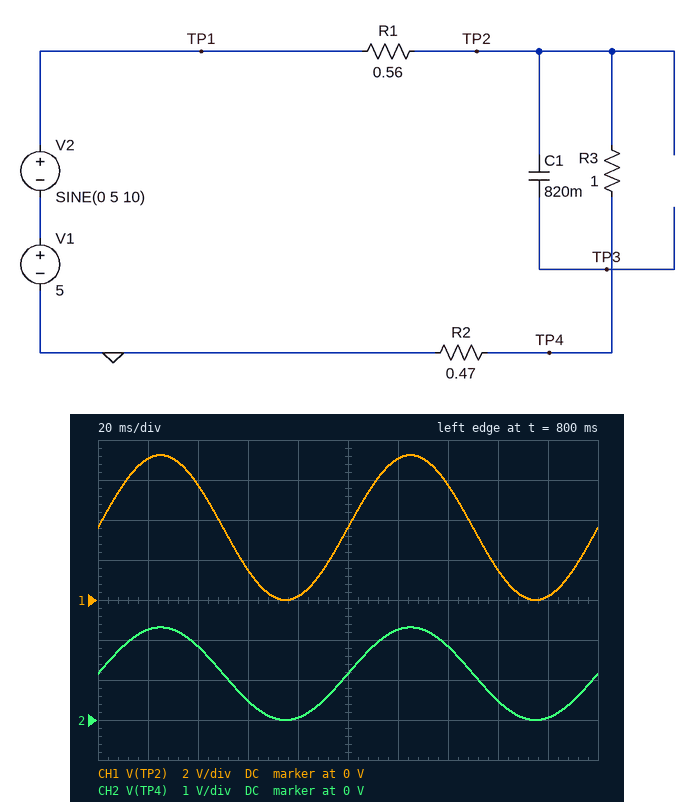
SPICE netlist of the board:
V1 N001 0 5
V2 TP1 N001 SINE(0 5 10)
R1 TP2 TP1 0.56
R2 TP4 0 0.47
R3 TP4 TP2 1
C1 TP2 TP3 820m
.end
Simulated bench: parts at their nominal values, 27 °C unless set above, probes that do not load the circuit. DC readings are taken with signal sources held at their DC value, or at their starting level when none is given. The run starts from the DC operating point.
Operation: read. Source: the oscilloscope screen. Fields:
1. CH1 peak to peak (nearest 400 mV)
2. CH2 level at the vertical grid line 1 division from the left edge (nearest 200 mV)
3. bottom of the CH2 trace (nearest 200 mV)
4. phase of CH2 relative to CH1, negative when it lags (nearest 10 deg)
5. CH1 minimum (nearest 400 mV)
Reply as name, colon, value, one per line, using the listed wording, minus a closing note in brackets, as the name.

CH1 peak to peak: 7.2 V
CH2 level at the vertical grid line 1 division from the left edge: 2.2 V
bottom of the CH2 trace: 0 V
phase of CH2 relative to CH1, negative when it lags: 0 deg
CH1 minimum: 0 V
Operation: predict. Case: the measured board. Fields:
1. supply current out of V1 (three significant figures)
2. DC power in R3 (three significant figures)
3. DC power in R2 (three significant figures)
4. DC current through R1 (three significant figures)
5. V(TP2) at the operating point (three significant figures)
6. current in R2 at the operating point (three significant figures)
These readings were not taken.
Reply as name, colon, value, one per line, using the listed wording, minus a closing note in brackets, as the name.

supply current out of V1: 2.46 A
DC power in R3: 6.07 W
DC power in R2: 2.85 W
DC current through R1: 2.46 A
V(TP2) at the operating point: 3.62 V
current in R2 at the operating point: 2.46 A
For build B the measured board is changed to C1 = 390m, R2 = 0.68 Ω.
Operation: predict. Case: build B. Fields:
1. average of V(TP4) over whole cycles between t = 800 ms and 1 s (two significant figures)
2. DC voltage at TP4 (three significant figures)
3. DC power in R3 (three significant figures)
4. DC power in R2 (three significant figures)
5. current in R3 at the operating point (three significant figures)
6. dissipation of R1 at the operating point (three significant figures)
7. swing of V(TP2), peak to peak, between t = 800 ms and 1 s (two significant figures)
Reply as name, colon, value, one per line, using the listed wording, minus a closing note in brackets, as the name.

average of V(TP4) over whole cycles between t = 800 ms and 1 s: 1.5 V
DC voltage at TP4: 1.52 V
DC power in R3: 4.98 W
DC power in R2: 3.39 W
current in R3 at the operating point: 2.23 A
dissipation of R1 at the operating point: 2.79 W
swing of V(TP2), peak to peak, between t = 800 ms and 1 s: 7.5 V
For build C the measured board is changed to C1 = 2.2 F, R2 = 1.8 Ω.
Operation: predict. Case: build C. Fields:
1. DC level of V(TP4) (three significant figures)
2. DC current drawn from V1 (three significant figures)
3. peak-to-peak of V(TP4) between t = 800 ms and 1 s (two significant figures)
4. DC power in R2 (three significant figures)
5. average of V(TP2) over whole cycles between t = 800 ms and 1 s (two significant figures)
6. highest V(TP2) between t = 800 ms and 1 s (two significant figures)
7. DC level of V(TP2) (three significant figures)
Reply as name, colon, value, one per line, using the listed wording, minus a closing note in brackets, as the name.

DC level of V(TP4): 2.68 V
DC current drawn from V1: 1.49 A
peak-to-peak of V(TP4) between t = 800 ms and 1 s: 5.4 V
DC power in R2: 3.99 W
average of V(TP2) over whole cycles between t = 800 ms and 1 s: 4.2 V
highest V(TP2) between t = 800 ms and 1 s: 8.3 V
DC level of V(TP2): 4.17 V
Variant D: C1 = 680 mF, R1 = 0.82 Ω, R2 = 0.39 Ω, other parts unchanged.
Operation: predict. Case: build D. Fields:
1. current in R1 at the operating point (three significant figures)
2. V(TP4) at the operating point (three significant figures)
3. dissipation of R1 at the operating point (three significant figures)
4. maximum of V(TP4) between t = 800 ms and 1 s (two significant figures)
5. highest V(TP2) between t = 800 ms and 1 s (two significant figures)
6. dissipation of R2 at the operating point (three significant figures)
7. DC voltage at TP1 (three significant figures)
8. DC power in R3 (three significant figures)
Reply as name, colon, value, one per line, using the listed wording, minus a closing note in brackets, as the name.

current in R1 at the operating point: 2.26 A
V(TP4) at the operating point: 882 mV
dissipation of R1 at the operating point: 4.20 W
maximum of V(TP4) between t = 800 ms and 1 s: 1.8 V
highest V(TP2) between t = 800 ms and 1 s: 6.3 V
dissipation of R2 at the operating point: 2.00 W
DC voltage at TP1: 5.00 V
DC power in R3: 5.12 W
